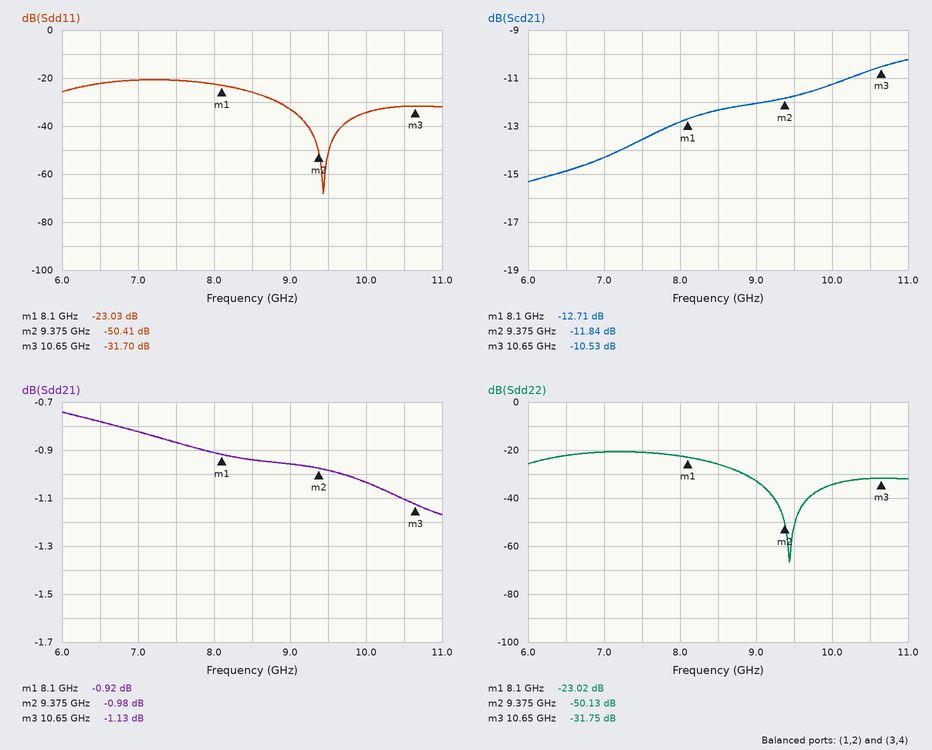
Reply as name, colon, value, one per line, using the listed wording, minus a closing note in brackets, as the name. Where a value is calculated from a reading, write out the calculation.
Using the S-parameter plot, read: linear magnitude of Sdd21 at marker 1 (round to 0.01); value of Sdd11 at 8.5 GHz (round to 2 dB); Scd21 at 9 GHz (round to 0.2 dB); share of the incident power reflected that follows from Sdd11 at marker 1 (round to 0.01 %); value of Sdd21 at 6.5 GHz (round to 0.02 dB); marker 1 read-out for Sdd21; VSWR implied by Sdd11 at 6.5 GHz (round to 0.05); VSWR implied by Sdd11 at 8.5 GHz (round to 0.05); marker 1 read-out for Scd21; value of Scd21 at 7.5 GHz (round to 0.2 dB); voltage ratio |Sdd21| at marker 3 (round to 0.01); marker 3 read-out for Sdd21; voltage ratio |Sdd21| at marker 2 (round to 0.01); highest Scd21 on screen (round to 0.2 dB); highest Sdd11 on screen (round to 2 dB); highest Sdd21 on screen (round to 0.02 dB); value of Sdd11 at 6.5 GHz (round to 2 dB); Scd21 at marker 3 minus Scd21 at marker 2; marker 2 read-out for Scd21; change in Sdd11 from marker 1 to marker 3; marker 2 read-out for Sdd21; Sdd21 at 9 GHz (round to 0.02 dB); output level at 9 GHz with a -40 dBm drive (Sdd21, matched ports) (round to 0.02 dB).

linear magnitude of Sdd21 at marker 1: 10^(-0.92/20) ≈ 0.90
value of Sdd11 at 8.5 GHz: -26 dB
Scd21 at 9 GHz: -12.0 dB
share of the incident power reflected that follows from Sdd11 at marker 1: 10^(-23.03/10) ≈ 0.50 %
value of Sdd21 at 6.5 GHz: -0.78 dB
marker 1 read-out for Sdd21: -0.92 dB
VSWR implied by Sdd11 at 6.5 GHz: |Γ| = 10^(-22/20) = 0.0794; VSWR = (1 + 0.0794)/(1 − 0.0794) ≈ 1.17, so 1.15 to the nearest 0.05
VSWR implied by Sdd11 at 8.5 GHz: |Γ| = 10^(-26/20) = 0.0501; VSWR = (1 + 0.0501)/(1 − 0.0501) ≈ 1.11, so 1.10 to the nearest 0.05
marker 1 read-out for Scd21: -12.71 dB
value of Scd21 at 7.5 GHz: -13.6 dB
voltage ratio |Sdd21| at marker 3: 10^(-1.13/20) ≈ 0.88
marker 3 read-out for Sdd21: -1.13 dB
voltage ratio |Sdd21| at marker 2: 10^(-0.98/20) ≈ 0.89
highest Scd21 on screen: -10.2 dB
highest Sdd11 on screen: -20 dB
highest Sdd21 on screen: -0.74 dB
value of Sdd11 at 6.5 GHz: -22 dB
Scd21 at marker 3 minus Scd21 at marker 2: -10.53 − (-11.84) = 1.31 dB
marker 2 read-out for Scd21: -11.84 dB
change in Sdd11 from marker 1 to marker 3: -31.7 − (-23.03) = -8.67 dB
marker 2 read-out for Sdd21: -0.98 dB
Sdd21 at 9 GHz: -0.96 dB
output level at 9 GHz with a -40 dBm drive (Sdd21, matched ports): -40 dBm + (-0.96 dB) = -40.96 dBm
